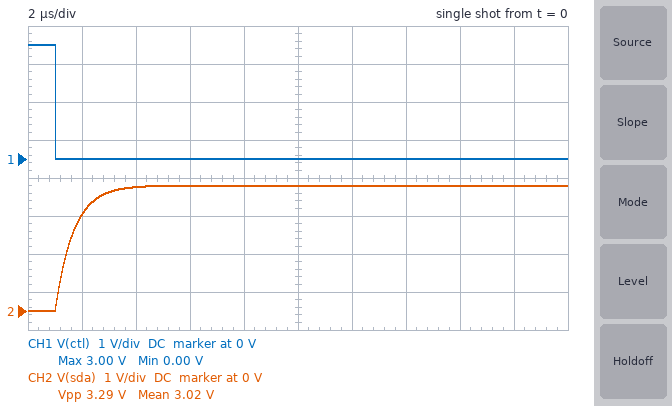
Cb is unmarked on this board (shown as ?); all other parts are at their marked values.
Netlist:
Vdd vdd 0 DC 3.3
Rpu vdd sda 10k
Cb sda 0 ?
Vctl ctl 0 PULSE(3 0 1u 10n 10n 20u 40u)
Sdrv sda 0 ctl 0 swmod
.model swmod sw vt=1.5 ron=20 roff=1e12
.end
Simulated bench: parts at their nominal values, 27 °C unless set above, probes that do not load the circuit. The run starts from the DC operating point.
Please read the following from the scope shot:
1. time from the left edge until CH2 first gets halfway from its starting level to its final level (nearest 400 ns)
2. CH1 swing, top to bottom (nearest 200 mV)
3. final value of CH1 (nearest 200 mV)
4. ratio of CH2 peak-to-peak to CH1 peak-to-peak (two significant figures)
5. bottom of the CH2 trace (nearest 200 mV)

1.6 µs
3.0 V
0 V
1.1
0 V
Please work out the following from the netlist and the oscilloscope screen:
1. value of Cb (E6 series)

68 pF
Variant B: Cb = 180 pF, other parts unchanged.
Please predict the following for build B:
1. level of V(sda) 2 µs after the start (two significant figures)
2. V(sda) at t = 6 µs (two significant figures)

1.4 V
3.1 V
